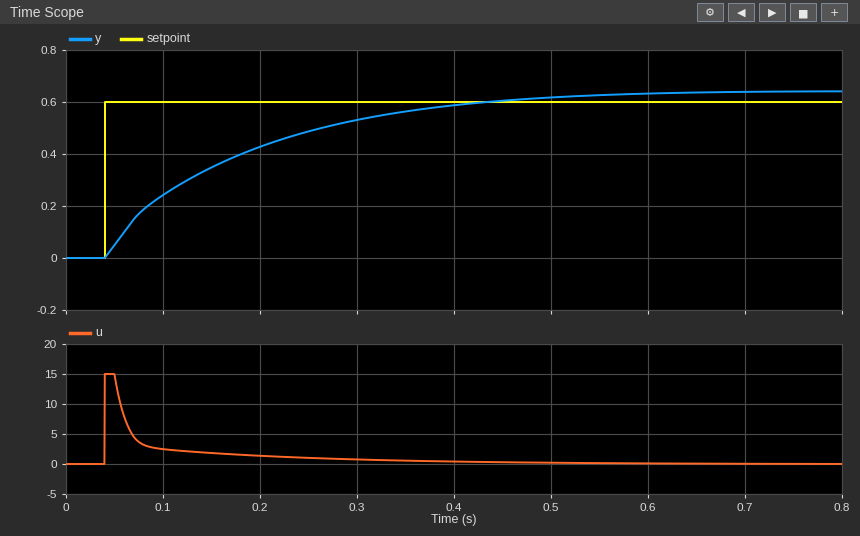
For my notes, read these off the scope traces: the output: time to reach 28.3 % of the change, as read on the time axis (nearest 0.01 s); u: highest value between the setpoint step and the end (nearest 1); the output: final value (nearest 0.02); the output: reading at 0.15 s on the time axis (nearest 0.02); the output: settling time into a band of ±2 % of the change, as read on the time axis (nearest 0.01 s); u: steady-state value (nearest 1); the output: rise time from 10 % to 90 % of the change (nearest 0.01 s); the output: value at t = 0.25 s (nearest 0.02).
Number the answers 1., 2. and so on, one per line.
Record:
1. 0.08 s
2. 15
3. 0.64
4. 0.34
5. 0.56 s
6. 0
7. 0.32 s
8. 0.48
